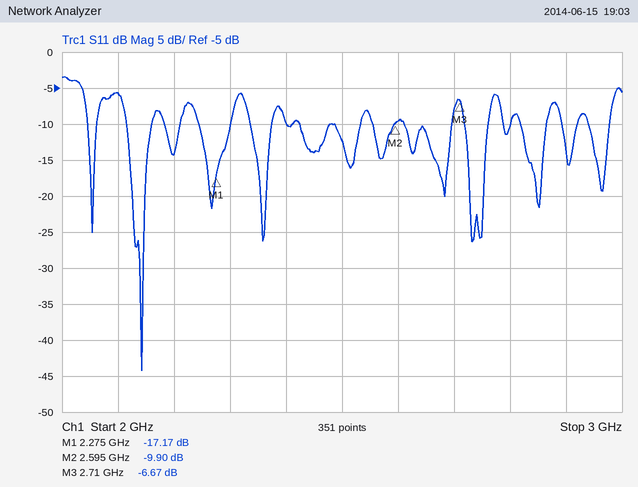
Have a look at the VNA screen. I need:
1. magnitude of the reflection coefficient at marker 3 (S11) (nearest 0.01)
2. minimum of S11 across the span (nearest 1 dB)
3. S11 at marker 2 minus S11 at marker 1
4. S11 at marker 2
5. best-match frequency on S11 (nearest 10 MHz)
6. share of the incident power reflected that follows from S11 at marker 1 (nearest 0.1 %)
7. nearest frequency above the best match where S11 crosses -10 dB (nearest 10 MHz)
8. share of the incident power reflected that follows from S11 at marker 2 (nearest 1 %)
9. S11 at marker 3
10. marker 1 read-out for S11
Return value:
0.46
-44 dB
7.27 dB
-9.90 dB
2.14 GHz
1.9 %
2.16 GHz
10 %
-6.67 dB
-17.17 dB
